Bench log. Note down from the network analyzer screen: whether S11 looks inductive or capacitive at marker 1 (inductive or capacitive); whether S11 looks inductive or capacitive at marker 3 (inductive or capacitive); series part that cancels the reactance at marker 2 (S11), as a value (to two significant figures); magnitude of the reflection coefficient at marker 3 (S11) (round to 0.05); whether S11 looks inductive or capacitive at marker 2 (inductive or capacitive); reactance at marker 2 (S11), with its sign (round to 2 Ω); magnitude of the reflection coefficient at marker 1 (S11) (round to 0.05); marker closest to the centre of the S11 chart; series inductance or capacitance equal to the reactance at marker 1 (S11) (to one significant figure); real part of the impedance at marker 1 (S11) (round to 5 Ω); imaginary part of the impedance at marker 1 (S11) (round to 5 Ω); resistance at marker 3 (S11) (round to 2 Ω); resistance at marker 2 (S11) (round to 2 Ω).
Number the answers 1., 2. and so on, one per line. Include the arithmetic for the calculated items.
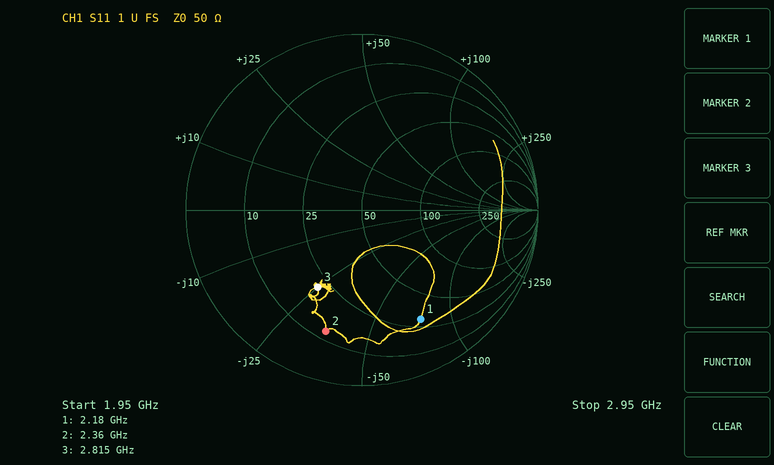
1. capacitive
2. capacitive
3. L = 36 Ω/(2π × 2.36 GHz) ≈ 2.4 nH
4. 0.50
5. capacitive
6. -36 Ω
7. 0.70
8. marker 3
9. C = 1/(2π × 2.18 GHz × 75 Ω) ≈ 1.0 pF
10. 30 Ω
11. -75 Ω
12. 22 Ω
13. 12 Ω
